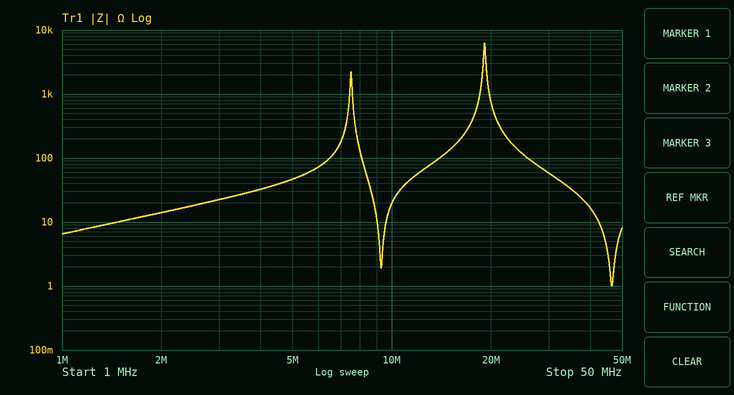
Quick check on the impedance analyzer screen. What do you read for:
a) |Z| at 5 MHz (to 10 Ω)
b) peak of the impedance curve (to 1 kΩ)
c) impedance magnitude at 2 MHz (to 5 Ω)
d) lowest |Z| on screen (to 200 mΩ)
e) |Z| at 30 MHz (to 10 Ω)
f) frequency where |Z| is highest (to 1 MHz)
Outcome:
50 Ω
6 kΩ
15 Ω
1.0 Ω
60 Ω
19 MHz
